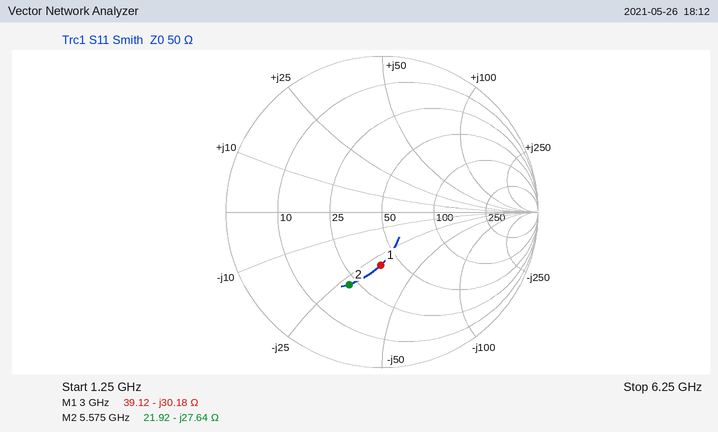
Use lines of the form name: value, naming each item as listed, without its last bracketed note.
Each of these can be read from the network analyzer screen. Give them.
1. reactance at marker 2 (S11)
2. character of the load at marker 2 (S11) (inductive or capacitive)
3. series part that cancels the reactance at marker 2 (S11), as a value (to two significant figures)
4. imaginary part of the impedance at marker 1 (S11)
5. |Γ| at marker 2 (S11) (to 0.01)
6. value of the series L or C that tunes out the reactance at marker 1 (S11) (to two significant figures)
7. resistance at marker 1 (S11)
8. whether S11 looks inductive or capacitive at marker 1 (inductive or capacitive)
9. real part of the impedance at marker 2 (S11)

reactance at marker 2: -27.64 Ω
character of the load at marker 2 (S11): capacitive
series part that cancels the reactance at marker 2 (S11), as a value: 790 pH
imaginary part of the impedance at marker 1: -30.18 Ω
|Γ| at marker 2 (S11): 0.51
value of the series L or C that tunes out the reactance at marker 1 (S11): 1.6 nH
resistance at marker 1: 39.12 Ω
whether S11 looks inductive or capacitive at marker 1: capacitive
real part of the impedance at marker 2: 21.92 Ω
